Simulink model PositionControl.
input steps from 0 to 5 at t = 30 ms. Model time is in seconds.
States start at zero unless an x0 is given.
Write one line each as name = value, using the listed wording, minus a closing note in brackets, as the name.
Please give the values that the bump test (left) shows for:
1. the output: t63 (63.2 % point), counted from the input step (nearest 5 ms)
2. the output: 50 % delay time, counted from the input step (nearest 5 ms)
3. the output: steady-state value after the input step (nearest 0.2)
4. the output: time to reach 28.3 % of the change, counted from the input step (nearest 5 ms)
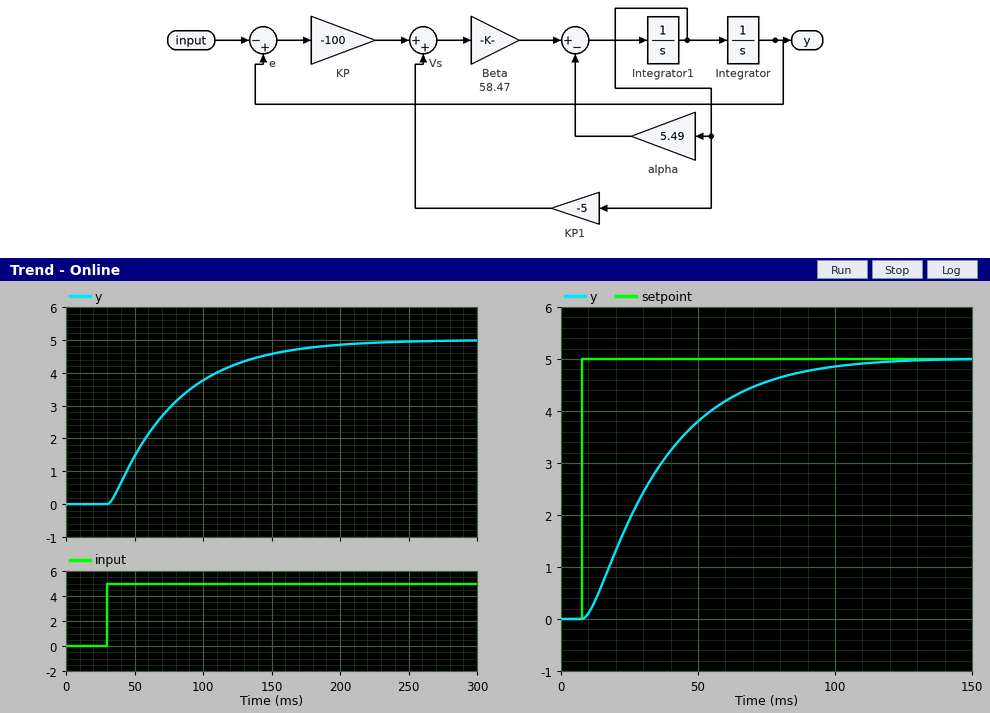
the output: t63 (63.2 % point), counted from the input step = 50 ms
the output: 50 % delay time, counted from the input step = 35 ms
the output: steady-state value after the input step = 5.0
the output: time to reach 28.3 % of the change, counted from the input step = 20 ms
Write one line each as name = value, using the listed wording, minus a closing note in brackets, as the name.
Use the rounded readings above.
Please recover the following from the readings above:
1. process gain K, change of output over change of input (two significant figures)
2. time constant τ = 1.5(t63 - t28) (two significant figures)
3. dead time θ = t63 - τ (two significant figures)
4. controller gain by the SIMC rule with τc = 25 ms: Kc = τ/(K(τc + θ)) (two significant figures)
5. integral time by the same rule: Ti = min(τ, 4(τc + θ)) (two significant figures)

process gain K, change of output over change of input = 1.0
time constant τ = 1.5(t63 - t28) = 45 ms
dead time θ = t63 - τ = 5.0 ms
controller gain by the SIMC rule with τc = 25 ms: Kc = τ/(K(τc + θ)) = 1.5
integral time by the same rule: Ti = min(τ, 4(τc + θ)) = 45 ms
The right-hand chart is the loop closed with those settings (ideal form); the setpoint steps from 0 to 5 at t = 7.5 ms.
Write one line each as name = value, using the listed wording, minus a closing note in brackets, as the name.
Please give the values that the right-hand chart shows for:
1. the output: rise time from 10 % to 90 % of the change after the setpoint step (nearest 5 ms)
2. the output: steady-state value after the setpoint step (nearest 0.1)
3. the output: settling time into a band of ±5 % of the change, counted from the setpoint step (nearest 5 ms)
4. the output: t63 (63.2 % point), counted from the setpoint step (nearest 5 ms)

the output: rise time from 10 % to 90 % of the change after the setpoint step = 60 ms
the output: steady-state value after the setpoint step = 5.0
the output: settling time into a band of ±5 % of the change, counted from the setpoint step = 80 ms
the output: t63 (63.2 % point), counted from the setpoint step = 30 ms
